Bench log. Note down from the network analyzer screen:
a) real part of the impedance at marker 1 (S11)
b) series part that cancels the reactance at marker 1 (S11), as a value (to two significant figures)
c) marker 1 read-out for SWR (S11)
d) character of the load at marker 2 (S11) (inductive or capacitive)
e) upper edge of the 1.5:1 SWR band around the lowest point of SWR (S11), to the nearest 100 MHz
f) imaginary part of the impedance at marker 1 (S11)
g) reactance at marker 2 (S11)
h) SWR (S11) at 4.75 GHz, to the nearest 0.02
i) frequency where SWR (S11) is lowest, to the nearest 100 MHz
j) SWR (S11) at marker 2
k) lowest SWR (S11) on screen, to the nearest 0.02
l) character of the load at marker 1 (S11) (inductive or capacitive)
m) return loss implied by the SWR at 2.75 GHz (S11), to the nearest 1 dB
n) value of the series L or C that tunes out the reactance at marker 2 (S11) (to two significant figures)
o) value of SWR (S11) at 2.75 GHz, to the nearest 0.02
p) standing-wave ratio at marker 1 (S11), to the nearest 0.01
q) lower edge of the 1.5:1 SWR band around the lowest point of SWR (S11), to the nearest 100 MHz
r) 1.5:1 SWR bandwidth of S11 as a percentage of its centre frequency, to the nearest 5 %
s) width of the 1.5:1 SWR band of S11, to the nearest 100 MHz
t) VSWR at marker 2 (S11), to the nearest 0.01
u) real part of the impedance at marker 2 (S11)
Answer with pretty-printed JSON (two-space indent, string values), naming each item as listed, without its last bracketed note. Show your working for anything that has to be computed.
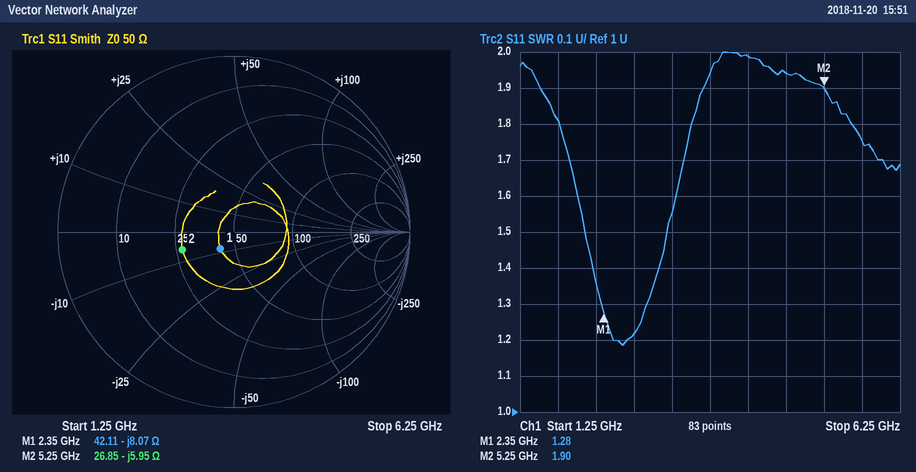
{
  "real part of the impedance at marker 1": "42.11 Ω",
  "series part that cancels the reactance at marker 1 (S11), as a value": "L = 8.07 Ω/(2π × 2.35 GHz) ≈ 547 pH, so 550 pH to two significant figures",
  "marker 1 read-out for SWR": "1.28",
  "character of the load at marker 2 (S11)": "capacitive",
  "upper edge of the 1.5:1 SWR band around the lowest point of SWR (S11), to the nearest 100 MHz": "3.2 GHz",
  "imaginary part of the impedance at marker 1": "-8.07 Ω",
  "reactance at marker 2": "-5.95 Ω",
  "SWR (S11) at 4.75 GHz, to the nearest 0.02": "1.94",
  "frequency where SWR (S11) is lowest, to the nearest 100 MHz": "2.6 GHz",
  "SWR (S11) at marker 2": "1.90",
  "lowest SWR (S11) on screen, to the nearest 0.02": "1.18",
  "character of the load at marker 1 (S11)": "capacitive",
  "return loss implied by the SWR at 2.75 GHz (S11), to the nearest 1 dB": "−20 log10((1.22 − 1)/(1.22 + 1)) ≈ 20 dB",
  "value of the series L or C that tunes out the reactance at marker 2 (S11)": "L = 5.95 Ω/(2π × 5.25 GHz) ≈ 180 pH",
  "value of SWR (S11) at 2.75 GHz, to the nearest 0.02": "1.22",
  "standing-wave ratio at marker 1 (S11), to the nearest 0.01": "1.28",
  "lower edge of the 1.5:1 SWR band around the lowest point of SWR (S11), to the nearest 100 MHz": "2.1 GHz",
  "1.5:1 SWR bandwidth of S11 as a percentage of its centre frequency, to the nearest 5 %": "1.1 GHz / 2.65 GHz ≈ 41.5 %, so 40 % to the nearest 5 %",
  "width of the 1.5:1 SWR band of S11, to the nearest 100 MHz": "3.2 GHz − 2.1 GHz = 1.1 GHz",
  "VSWR at marker 2 (S11), to the nearest 0.01": "1.90",
  "real part of the impedance at marker 2": "26.85 Ω"
}
